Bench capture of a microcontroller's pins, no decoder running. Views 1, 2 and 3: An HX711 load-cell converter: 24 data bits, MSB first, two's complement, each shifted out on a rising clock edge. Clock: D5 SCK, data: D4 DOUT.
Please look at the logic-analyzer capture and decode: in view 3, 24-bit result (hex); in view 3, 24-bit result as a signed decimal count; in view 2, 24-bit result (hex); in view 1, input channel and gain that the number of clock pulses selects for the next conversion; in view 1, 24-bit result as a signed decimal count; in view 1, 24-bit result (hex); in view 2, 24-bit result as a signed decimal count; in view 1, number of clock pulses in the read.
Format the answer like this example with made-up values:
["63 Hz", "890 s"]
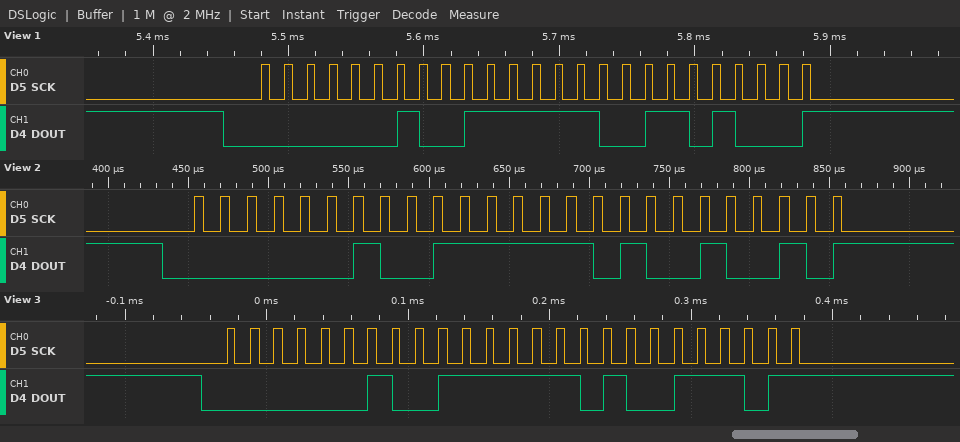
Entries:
["0x027E9D", "163485", "0x027E92", "channel A, gain 128", "163432", "0x027E68", "163474", "25"]
